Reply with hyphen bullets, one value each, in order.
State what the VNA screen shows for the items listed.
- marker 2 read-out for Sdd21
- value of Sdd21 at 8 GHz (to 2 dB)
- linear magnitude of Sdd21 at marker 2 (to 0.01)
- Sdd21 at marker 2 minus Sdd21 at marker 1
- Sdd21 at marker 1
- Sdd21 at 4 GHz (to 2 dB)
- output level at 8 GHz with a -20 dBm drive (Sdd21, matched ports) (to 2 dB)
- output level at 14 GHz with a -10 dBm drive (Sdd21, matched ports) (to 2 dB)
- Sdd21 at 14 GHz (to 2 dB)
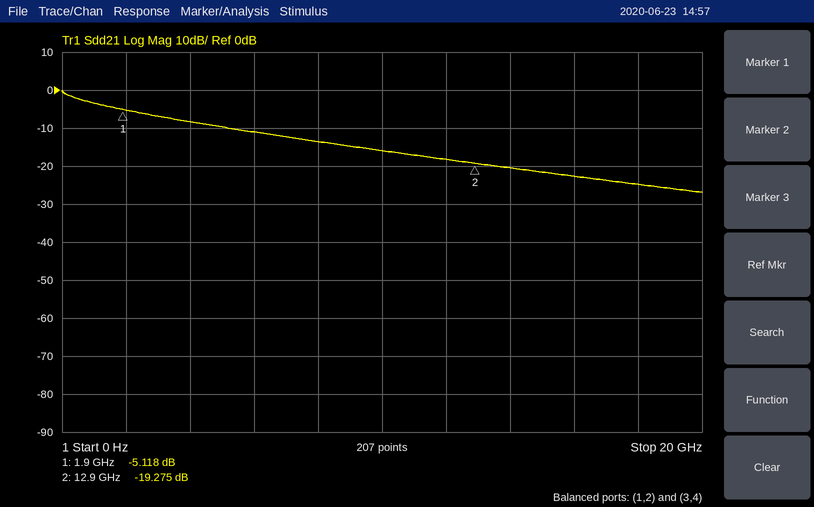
- -19.275 dB
- -14 dB
- 0.11
- -14.157 dB
- -5.118 dB
- -8 dB
- -34 dBm
- -30 dBm
- -20 dB
